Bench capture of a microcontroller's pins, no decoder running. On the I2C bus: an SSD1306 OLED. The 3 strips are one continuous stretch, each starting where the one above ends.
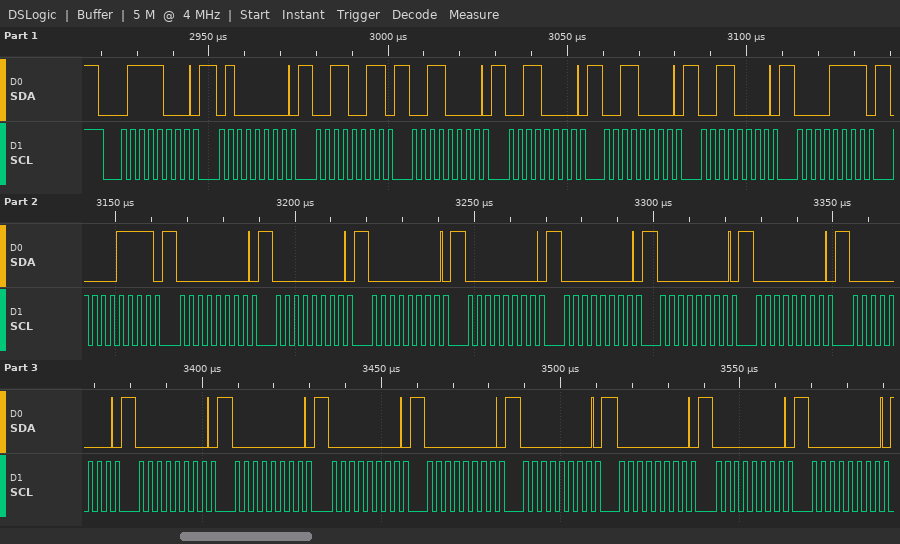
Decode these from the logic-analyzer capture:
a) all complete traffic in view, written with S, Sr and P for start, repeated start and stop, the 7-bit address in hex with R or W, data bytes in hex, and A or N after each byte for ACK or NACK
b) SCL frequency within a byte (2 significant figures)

S 3CW A 40 A 33 A 30 A 30 A 30 A 30 A 0F A 0F A 00 A 00 A 00 A 00 A 00 A 00 A 00 A 00 A 00 A 00 A 00 A 00 A 00 A 00 A 00 A 00 A
400 kHz
